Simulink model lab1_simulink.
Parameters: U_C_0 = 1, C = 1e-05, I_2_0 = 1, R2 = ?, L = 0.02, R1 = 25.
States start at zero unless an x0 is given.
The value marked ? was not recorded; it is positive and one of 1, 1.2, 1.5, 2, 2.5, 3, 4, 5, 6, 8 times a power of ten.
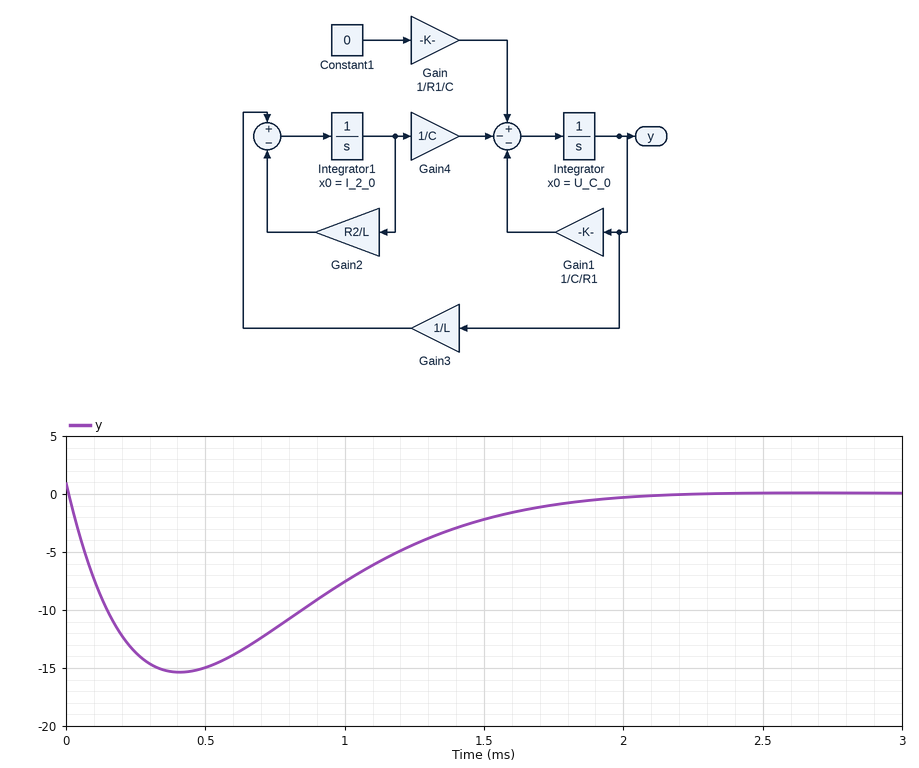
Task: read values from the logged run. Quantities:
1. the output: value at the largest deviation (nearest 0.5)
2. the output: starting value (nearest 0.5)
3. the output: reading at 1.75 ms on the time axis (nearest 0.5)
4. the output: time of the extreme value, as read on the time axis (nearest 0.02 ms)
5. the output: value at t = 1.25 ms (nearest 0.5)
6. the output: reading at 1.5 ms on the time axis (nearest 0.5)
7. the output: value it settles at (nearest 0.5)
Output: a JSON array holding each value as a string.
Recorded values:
["-15.5", "1.0", "-1.0", "0.40 ms", "-4.5", "-2.0", "0.0"]
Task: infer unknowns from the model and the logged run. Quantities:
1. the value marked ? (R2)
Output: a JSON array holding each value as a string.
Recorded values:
["10"]
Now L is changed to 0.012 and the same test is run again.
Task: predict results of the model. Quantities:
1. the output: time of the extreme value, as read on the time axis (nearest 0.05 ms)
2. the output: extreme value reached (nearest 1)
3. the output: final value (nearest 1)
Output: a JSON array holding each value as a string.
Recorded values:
["0.35 ms", "-13", "0"]
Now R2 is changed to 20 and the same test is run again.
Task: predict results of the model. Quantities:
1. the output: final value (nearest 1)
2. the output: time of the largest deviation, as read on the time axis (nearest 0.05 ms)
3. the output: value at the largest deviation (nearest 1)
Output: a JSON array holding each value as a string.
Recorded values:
["0", "0.35 ms", "-14"]
